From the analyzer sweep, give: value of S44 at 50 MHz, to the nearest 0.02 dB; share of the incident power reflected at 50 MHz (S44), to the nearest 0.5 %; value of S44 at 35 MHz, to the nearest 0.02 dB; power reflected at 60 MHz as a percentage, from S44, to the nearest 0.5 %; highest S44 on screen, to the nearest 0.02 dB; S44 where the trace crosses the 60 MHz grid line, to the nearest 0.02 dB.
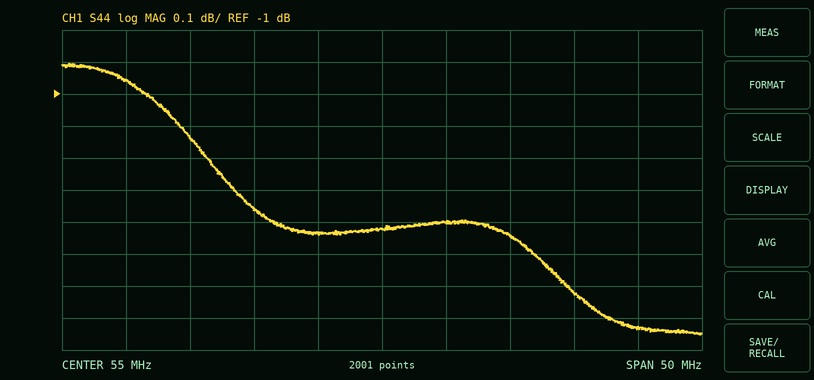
-1.44 dB
72.0 %
-0.96 dB
72.5 %
-0.90 dB
-1.40 dB
